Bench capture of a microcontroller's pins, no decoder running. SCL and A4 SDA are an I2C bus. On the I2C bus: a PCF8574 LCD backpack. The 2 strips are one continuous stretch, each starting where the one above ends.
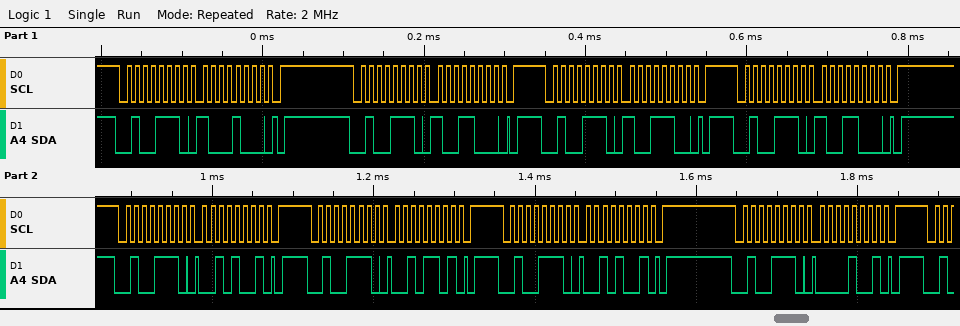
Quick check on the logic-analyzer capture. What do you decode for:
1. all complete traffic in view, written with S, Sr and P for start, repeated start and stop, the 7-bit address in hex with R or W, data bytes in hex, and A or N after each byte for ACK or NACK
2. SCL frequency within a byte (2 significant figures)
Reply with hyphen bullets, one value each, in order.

- S 27W A 88 A P S 27W A 98 A P S 27W A 9C A P S 27W A 98 A P S 27W A 29 A P S 27W A 2D A P S 27W A 29 A P S 27W A 09 A P
- 100 kHz
